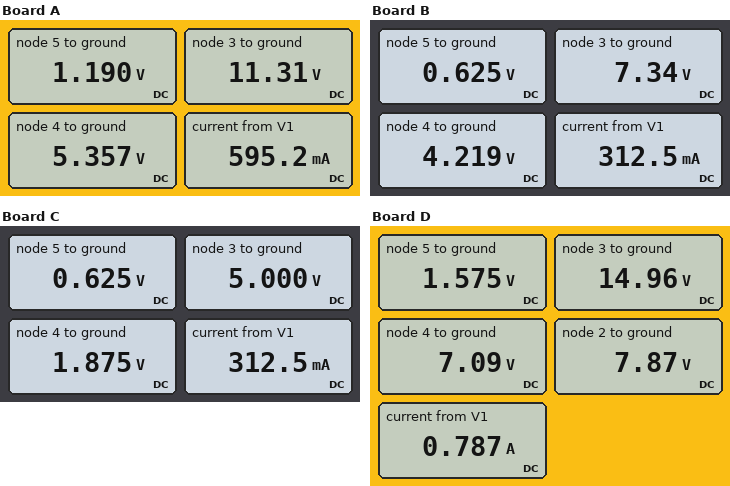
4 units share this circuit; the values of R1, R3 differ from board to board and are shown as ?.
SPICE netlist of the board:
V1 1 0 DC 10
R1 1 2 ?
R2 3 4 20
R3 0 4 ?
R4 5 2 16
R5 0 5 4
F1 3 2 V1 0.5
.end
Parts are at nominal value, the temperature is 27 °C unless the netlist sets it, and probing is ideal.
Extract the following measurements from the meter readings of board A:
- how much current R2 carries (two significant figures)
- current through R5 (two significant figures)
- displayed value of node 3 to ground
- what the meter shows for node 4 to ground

300 mA
300 mA
11.31 V
5.357 V
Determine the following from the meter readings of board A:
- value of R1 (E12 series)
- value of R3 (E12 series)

6.8 Ω
18 Ω
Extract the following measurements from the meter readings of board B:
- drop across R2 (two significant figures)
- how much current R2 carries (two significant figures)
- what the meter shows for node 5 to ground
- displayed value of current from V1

3.1 V
160 mA
0.625 V
312.5 mA
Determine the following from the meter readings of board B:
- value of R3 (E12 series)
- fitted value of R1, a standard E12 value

27 Ω
22 Ω
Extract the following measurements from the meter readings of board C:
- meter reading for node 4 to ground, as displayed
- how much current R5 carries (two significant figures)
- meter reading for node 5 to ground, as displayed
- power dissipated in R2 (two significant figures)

1.875 V
160 mA
0.625 V
490 mW
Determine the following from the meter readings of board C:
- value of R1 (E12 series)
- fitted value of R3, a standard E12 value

22 Ω
12 Ω
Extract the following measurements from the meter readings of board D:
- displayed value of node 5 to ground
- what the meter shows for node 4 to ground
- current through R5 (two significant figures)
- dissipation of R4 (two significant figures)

1.575 V
7.09 V
390 mA
2.5 W
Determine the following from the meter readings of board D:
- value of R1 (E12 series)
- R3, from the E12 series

2.7 Ω
18 Ω
